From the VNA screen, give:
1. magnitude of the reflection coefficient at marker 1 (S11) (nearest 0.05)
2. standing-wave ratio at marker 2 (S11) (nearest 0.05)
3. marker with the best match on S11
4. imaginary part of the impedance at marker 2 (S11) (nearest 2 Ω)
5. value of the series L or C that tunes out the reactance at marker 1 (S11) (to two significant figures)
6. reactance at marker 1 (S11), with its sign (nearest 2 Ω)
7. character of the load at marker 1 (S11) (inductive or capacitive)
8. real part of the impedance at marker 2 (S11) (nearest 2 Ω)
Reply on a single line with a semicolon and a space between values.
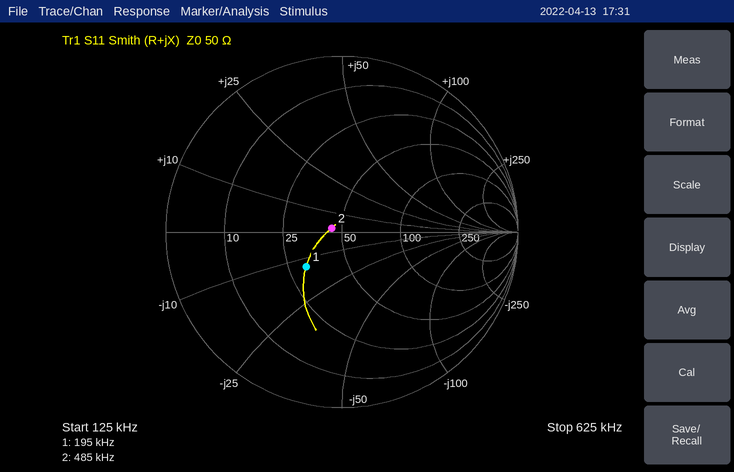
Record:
0.30; 1.15; marker 2; +2 Ω; 11 µH; -14 Ω; capacitive; 44 Ω
